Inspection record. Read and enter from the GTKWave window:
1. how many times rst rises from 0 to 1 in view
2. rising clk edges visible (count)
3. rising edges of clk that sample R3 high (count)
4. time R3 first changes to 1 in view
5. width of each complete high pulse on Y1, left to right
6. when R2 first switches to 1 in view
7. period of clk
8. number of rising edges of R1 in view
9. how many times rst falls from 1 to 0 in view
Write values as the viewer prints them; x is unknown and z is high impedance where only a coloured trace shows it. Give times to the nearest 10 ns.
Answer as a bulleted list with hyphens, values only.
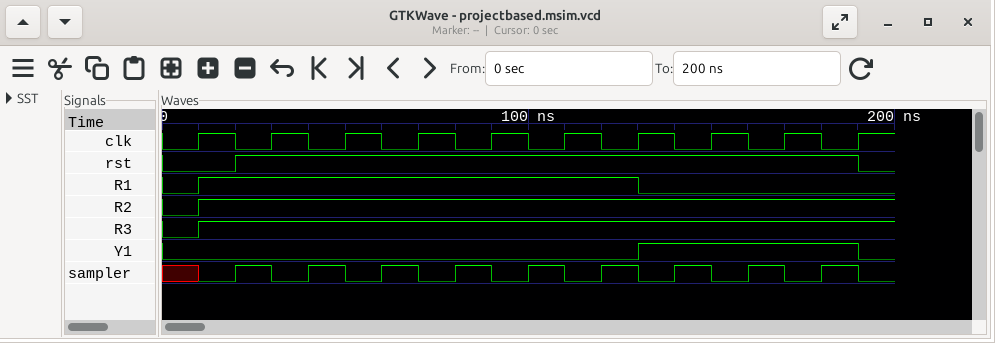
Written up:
- 1
- 10
- 9
- 10 ns
- 60 ns
- 10 ns
- 20 ns
- 1
- 1
